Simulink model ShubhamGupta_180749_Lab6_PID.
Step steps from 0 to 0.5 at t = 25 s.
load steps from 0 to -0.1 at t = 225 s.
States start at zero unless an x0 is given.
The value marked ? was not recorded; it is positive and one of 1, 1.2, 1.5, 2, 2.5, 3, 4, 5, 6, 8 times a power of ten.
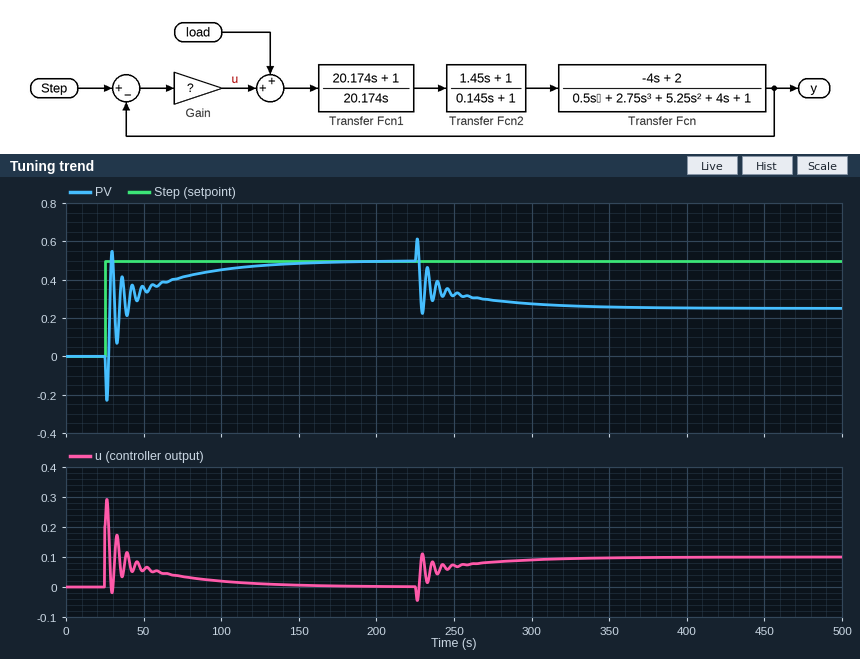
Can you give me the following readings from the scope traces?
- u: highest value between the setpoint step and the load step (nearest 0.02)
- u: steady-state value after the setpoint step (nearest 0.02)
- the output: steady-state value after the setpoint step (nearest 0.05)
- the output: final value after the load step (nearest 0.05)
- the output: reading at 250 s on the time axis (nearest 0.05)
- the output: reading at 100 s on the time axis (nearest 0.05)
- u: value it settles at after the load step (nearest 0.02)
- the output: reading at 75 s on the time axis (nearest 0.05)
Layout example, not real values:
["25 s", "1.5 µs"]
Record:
["0.30", "0.00", "0.50", "0.25", "0.30", "0.45", "0.10", "0.40"]
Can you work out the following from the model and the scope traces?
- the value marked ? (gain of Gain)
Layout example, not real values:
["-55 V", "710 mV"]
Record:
["0.4"]
